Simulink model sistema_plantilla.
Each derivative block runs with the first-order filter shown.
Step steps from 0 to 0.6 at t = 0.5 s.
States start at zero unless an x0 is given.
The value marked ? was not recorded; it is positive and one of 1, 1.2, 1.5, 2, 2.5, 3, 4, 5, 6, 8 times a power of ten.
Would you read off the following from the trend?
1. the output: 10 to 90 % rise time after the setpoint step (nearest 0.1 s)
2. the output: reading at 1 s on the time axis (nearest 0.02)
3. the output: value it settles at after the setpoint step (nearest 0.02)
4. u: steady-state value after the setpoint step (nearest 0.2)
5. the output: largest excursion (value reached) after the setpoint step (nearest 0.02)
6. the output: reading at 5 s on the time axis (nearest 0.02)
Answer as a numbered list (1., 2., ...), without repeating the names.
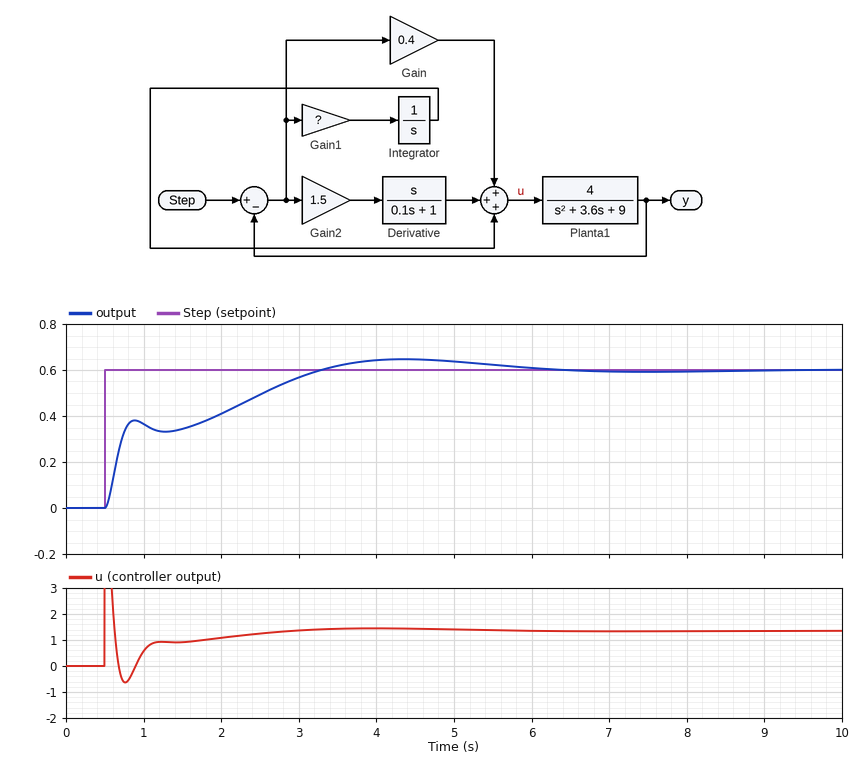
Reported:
1. 2.2 s
2. 0.36
3. 0.60
4. 1.4
5. 0.64
6. 0.64
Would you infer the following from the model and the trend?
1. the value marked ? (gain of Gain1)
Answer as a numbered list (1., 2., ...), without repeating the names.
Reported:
1. 3
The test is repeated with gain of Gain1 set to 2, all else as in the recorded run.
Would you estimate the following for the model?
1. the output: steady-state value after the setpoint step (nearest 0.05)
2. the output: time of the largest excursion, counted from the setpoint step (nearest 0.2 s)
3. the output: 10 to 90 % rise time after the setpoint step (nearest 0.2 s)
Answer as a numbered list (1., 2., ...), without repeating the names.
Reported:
1. 0.60
2. 5.2 s
3. 3.0 s
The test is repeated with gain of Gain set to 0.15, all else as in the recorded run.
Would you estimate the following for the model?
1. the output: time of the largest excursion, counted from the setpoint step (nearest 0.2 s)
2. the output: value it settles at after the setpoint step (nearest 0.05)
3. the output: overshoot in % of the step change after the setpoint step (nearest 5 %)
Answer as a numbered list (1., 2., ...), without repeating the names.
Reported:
1. 3.8 s
2. 0.60
3. 10 %
